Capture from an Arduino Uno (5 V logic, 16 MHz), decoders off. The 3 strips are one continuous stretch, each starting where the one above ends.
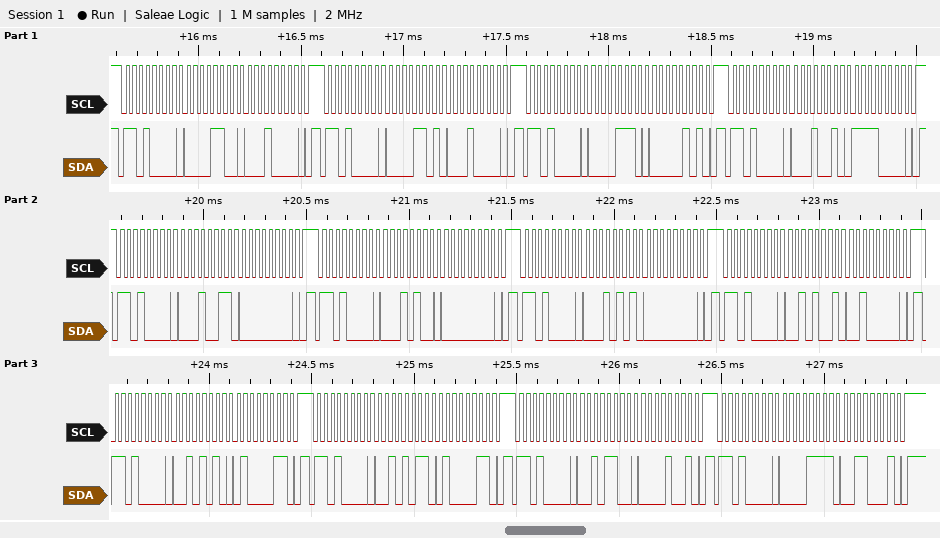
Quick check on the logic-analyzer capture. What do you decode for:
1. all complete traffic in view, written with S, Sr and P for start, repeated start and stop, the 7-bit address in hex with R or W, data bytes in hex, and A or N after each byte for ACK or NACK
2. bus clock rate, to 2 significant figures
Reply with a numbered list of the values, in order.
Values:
1. S 68W A 0C A 10 A P S 68W A 0D A 10 A P S 68W A 0E A 05 A P S 68W A 12 A F0 A P S 68W A 13 A 00 A P S 68W A 14 A 00 A P S 68W A 15 A 00 A P S 68W A 29 A 20 A P S 68W A 2A A 43 A P S 68W A 2B A 43 A P S 68W A 2C A 09 A P S 68W A 0F A 31 A P
2. 31 kHz
